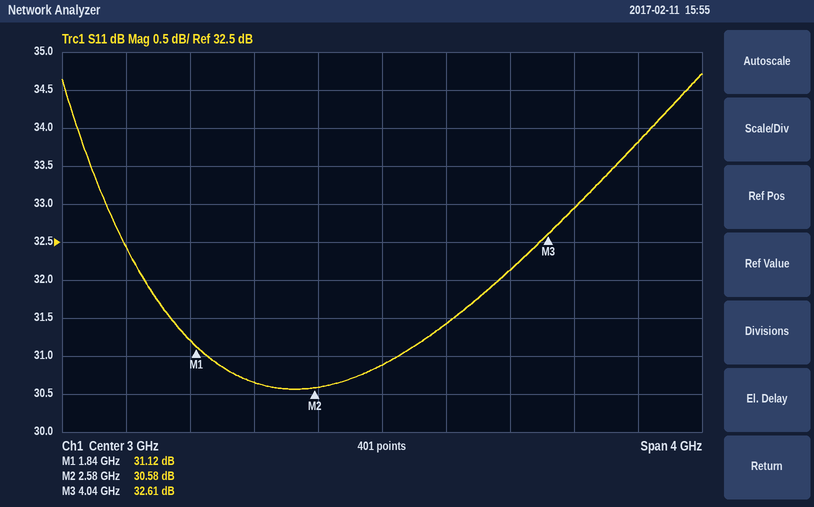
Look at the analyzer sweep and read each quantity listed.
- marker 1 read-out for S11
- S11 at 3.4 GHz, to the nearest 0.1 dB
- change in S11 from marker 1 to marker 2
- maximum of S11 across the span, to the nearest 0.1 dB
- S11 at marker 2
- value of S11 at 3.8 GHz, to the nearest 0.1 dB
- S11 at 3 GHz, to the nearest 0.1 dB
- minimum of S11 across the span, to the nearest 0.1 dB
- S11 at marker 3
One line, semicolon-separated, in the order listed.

31.12 dB; 31.4 dB; -0.54 dB; 34.7 dB; 30.58 dB; 32.1 dB; 30.9 dB; 30.6 dB; 32.61 dB
